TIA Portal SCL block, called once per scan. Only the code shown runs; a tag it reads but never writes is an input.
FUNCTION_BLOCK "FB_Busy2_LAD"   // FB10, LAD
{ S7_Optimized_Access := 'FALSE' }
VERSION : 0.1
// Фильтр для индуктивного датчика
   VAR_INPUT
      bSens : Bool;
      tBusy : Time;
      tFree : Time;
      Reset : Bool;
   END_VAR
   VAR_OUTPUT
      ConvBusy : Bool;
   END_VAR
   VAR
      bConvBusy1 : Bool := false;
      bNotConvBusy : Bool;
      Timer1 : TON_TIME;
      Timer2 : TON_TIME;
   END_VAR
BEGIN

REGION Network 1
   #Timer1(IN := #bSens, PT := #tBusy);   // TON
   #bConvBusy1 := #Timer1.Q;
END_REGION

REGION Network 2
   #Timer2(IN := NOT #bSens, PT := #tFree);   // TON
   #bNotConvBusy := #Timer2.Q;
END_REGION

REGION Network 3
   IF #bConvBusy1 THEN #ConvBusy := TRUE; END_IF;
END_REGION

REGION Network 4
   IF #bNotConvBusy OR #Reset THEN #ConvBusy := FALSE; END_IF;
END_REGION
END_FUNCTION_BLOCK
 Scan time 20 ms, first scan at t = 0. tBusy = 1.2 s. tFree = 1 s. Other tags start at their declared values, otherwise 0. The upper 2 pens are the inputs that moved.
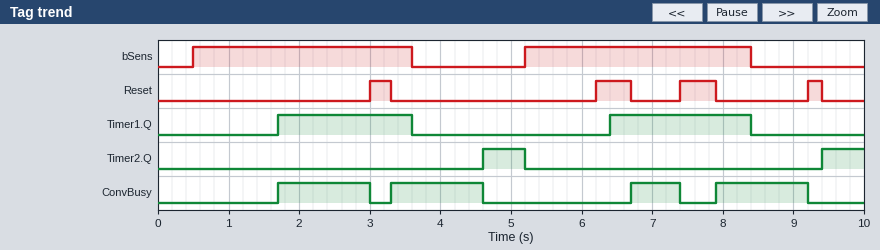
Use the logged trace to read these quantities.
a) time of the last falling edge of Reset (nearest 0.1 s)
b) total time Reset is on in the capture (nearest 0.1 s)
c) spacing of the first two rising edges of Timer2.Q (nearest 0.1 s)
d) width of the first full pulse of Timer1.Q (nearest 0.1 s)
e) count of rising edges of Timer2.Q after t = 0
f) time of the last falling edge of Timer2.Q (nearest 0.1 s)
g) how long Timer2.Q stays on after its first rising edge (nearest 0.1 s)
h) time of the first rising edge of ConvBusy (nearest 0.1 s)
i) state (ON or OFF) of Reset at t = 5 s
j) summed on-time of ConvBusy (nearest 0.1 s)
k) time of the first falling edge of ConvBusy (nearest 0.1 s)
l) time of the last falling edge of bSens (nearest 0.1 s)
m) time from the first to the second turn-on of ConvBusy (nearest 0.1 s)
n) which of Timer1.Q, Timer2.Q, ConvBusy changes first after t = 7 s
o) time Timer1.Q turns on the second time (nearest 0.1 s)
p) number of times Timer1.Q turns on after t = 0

9.4 s
1.5 s
4.8 s
1.9 s
2
5.2 s
0.6 s
1.7 s
OFF
4.6 s
3.0 s
8.4 s
1.6 s
ConvBusy
6.4 s
2
